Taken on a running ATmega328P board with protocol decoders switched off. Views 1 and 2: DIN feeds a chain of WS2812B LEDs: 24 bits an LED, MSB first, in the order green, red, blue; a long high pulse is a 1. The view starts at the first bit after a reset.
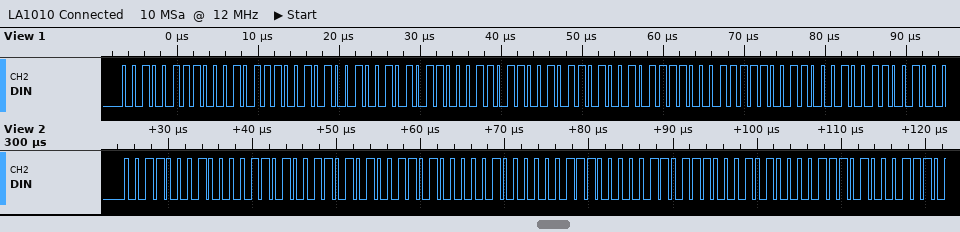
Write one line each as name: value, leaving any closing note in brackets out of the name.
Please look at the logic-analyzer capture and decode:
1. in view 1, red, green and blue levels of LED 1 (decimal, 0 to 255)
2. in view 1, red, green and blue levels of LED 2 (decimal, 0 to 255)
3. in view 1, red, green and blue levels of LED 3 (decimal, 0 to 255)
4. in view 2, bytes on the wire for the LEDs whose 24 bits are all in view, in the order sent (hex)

in view 1, red, green and blue levels of LED 1: 23, 39, 41
in view 1, red, green and blue levels of LED 2: 27, 43, 45
in view 1, red, green and blue levels of LED 3: 31, 47, 49
in view 2, bytes on the wire for the LEDs whose 24 bits are all in view, in the order sent: 31 0D 35 34 10 38 37 14 3A
